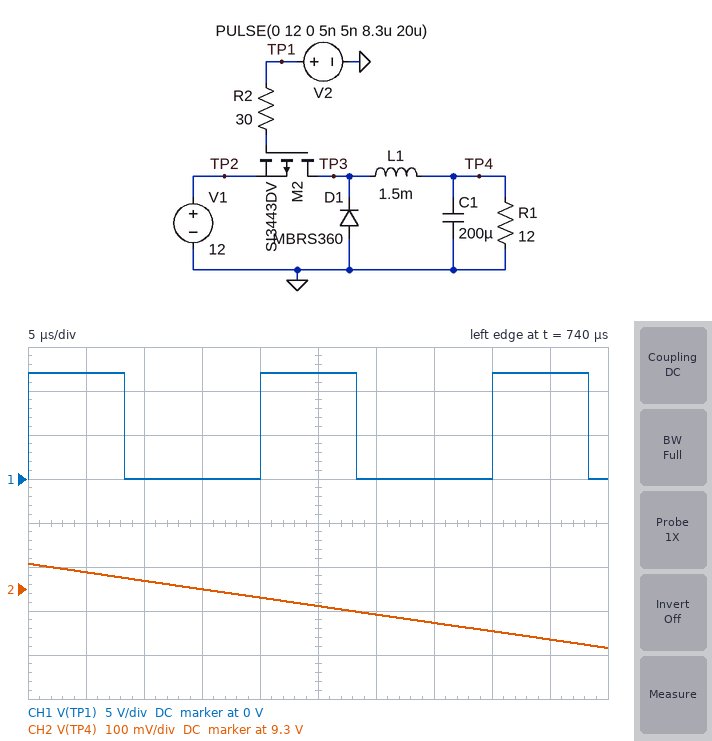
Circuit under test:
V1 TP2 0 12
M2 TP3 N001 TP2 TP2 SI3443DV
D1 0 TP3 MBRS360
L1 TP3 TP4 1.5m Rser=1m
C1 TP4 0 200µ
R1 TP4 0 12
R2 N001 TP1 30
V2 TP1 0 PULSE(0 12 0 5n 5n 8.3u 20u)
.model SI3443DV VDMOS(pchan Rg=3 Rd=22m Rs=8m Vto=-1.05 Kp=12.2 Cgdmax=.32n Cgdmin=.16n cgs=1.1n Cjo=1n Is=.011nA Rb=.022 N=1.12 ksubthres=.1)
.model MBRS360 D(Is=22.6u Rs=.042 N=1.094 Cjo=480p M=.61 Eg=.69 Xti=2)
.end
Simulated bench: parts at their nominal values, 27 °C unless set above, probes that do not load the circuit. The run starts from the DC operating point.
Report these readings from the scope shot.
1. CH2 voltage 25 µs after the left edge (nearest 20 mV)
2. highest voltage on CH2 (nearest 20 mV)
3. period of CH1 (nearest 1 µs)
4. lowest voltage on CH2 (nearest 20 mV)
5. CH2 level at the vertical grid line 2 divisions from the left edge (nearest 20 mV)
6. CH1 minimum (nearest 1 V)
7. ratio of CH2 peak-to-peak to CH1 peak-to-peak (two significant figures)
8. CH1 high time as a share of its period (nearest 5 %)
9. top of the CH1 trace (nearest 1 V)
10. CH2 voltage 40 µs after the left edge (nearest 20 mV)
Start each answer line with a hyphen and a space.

- 9.26 V
- 9.36 V
- 20 µs
- 9.16 V
- 9.32 V
- 0 V
- 0.016
- 40 %
- 12 V
- 9.20 V
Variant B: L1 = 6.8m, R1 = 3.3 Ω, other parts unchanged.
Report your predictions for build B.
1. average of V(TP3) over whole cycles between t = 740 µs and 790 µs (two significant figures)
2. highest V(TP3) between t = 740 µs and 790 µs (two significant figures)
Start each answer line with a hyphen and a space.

- 6.8 V
- 12 V
